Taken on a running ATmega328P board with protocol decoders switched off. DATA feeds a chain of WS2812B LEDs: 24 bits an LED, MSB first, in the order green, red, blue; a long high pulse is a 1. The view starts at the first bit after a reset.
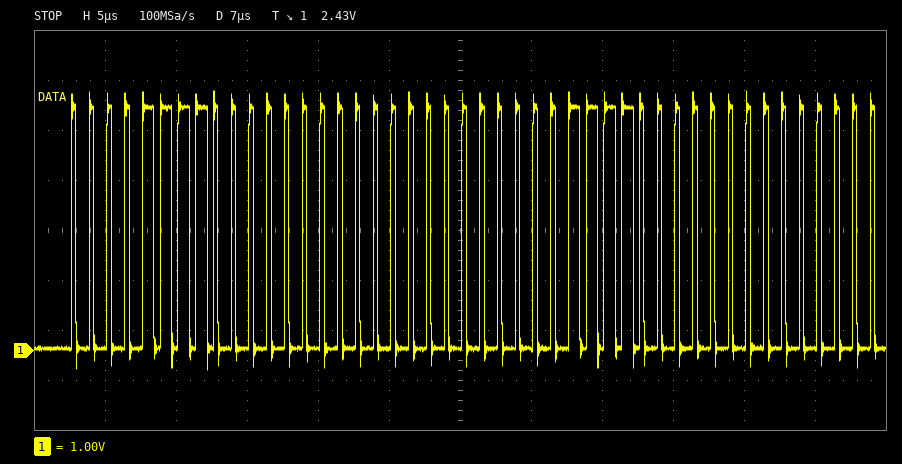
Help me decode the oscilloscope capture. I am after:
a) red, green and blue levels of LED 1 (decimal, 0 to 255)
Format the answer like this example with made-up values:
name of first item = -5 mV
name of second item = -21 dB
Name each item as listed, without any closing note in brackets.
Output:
red, green and blue levels of LED 1 = 0, 15, 0
